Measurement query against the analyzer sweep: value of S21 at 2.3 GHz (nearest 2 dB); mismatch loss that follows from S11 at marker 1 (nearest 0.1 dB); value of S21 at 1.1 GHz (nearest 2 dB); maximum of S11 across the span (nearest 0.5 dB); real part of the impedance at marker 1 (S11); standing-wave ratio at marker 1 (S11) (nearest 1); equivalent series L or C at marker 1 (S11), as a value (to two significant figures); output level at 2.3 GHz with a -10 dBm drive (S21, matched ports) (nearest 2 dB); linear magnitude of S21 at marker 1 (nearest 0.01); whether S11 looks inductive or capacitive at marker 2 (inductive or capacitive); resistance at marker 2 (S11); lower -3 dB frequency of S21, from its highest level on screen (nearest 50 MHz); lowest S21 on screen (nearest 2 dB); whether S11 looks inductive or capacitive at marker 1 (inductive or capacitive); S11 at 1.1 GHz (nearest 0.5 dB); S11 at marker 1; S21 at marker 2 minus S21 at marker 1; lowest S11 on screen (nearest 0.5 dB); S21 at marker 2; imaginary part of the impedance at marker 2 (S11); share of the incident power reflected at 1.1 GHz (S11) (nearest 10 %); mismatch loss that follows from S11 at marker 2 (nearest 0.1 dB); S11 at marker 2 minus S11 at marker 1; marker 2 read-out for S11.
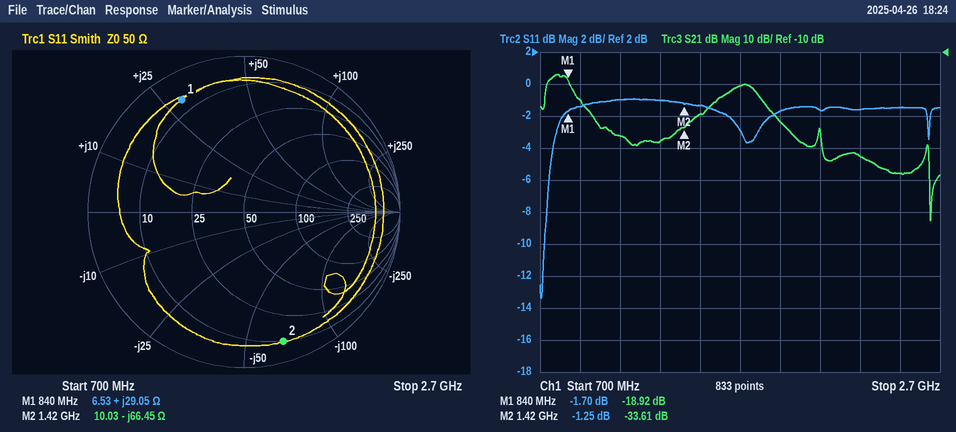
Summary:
-42 dB
4.9 dB
-36 dB
-1.0 dB
6.53 Ω
10
5.5 nH
-52 dBm
0.11
capacitive
10.03 Ω
750 MHz
-62 dB
inductive
-1.0 dB
-1.70 dB
-14.69 dB
-13.5 dB
-33.61 dB
-66.45 Ω
80 %
6.0 dB
0.45 dB
-1.25 dB
